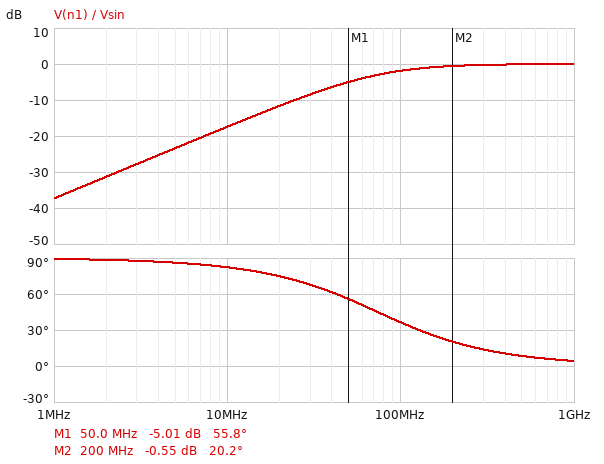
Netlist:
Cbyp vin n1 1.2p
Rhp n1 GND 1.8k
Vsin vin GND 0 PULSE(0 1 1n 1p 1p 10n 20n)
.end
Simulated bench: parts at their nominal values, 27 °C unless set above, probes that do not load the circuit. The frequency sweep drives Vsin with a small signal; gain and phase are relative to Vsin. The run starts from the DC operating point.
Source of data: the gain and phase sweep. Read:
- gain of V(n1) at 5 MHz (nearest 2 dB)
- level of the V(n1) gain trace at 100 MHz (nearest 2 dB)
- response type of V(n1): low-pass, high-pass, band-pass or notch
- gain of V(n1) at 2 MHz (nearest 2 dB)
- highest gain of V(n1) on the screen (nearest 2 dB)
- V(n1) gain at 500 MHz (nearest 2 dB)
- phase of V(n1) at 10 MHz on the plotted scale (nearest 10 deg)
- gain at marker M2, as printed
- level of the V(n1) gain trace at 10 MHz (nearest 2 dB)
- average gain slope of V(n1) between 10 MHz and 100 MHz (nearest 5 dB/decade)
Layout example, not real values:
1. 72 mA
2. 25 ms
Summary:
1. -24 dB
2. -2 dB
3. high-pass
4. -32 dB
5. 0 dB
6. 0 dB
7. 80 deg
8. -0.55 dB
9. -18 dB
10. 15 dB/decade
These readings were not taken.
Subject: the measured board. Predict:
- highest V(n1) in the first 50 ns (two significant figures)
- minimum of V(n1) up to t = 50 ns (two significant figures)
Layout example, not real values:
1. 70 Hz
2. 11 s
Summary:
1. 1.0 V
2. -990 mV
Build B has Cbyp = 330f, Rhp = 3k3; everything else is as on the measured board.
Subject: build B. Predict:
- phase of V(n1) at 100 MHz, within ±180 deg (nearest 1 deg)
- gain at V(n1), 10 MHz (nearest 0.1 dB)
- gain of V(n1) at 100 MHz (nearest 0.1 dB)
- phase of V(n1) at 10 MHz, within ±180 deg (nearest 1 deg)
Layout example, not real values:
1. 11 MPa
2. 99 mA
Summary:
1. 56 deg
2. -23.3 dB
3. -5.0 dB
4. 86 deg
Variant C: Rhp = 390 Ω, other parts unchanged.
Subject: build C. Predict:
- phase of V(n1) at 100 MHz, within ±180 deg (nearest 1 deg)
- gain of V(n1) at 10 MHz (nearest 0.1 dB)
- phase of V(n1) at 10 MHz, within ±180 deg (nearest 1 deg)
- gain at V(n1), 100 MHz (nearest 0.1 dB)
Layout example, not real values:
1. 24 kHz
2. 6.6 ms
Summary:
1. 74 deg
2. -30.6 dB
3. 88 deg
4. -11.0 dB
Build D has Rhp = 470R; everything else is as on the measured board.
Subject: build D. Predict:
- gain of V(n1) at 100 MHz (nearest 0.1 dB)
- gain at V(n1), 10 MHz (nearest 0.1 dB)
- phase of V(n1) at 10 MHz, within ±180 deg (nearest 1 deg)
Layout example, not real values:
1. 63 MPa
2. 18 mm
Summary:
1. -9.5 dB
2. -29.0 dB
3. 88 deg
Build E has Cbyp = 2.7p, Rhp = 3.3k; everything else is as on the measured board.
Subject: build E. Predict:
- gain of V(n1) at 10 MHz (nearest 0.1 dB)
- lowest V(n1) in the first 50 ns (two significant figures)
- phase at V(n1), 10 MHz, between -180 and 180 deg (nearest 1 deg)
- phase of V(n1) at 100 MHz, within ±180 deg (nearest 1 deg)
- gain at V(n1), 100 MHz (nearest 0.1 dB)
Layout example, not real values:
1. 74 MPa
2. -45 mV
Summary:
1. -6.2 dB
2. -750 mV
3. 61 deg
4. 10 deg
5. -0.1 dB
